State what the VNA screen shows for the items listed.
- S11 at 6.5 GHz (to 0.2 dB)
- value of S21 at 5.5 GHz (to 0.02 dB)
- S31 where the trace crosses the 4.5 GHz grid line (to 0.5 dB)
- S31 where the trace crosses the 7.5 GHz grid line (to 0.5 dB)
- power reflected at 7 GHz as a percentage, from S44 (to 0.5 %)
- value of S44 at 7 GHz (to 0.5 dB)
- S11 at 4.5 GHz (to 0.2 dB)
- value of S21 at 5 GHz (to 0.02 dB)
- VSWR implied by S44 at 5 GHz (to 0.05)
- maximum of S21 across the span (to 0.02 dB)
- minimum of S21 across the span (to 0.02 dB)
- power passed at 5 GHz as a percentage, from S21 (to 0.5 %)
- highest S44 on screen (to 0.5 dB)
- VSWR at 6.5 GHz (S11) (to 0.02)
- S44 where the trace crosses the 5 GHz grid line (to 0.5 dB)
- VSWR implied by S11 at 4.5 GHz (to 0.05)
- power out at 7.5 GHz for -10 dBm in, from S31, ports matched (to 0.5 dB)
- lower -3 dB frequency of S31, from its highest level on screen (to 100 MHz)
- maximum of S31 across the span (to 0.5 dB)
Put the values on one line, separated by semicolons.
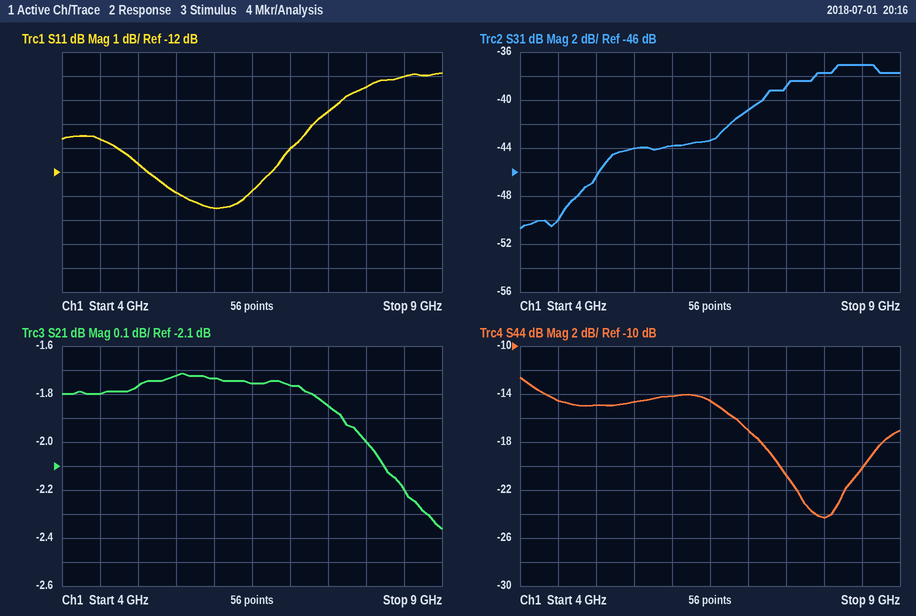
-12.8 dB; -1.72 dB; -50.0 dB; -39.0 dB; 2.0 %; -17.0 dB; -10.6 dB; -1.76 dB; 1.45; -1.72 dB; -2.36 dB; 66.5 %; -12.5 dB; 1.60; -15.0 dB; 1.85; -49.0 dBm; 7.2 GHz; -37.0 dB
